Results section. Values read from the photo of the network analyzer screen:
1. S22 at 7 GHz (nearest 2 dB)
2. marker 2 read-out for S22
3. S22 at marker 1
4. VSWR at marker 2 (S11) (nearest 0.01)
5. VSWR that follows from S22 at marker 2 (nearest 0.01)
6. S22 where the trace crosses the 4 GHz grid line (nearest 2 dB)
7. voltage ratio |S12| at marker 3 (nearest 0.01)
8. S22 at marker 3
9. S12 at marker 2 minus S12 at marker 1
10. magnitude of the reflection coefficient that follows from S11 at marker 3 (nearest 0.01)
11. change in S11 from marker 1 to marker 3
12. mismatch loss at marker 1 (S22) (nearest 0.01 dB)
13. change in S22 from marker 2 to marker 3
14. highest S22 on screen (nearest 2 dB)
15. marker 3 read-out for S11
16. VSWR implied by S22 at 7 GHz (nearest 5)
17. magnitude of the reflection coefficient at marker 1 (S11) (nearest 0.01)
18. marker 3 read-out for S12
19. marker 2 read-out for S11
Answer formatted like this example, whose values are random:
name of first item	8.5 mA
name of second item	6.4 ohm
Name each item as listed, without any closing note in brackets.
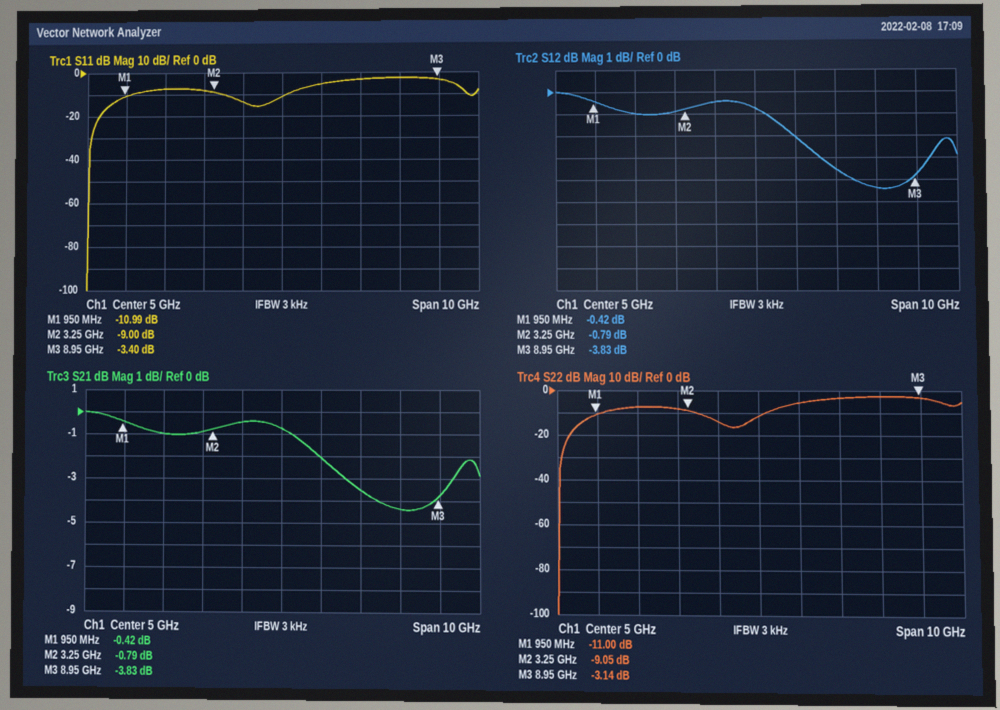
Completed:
S22 at 7 GHz	-4 dB
marker 2 read-out for S22	-9.05 dB
S22 at marker 1	-11.00 dB
VSWR at marker 2 (S11)	2.10
VSWR that follows from S22 at marker 2	2.09
S22 where the trace crosses the 4 GHz grid line	-14 dB
voltage ratio |S12| at marker 3	0.64
S22 at marker 3	-3.14 dB
S12 at marker 2 minus S12 at marker 1	-0.37 dB
magnitude of the reflection coefficient that follows from S11 at marker 3	0.68
change in S11 from marker 1 to marker 3	7.59 dB
mismatch loss at marker 1 (S22)	0.36 dB
change in S22 from marker 2 to marker 3	5.91 dB
highest S22 on screen	-2 dB
marker 3 read-out for S11	-3.40 dB
VSWR implied by S22 at 7 GHz	5
magnitude of the reflection coefficient at marker 1 (S11)	0.28
marker 3 read-out for S12	-3.83 dB
marker 2 read-out for S11	-9.00 dB
